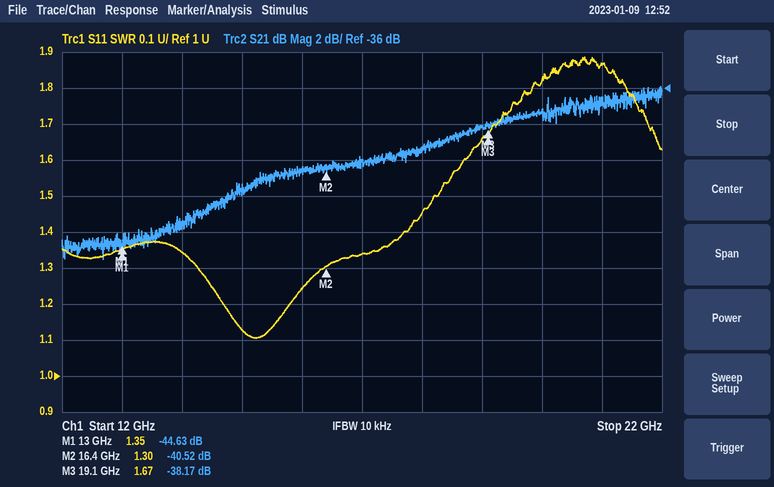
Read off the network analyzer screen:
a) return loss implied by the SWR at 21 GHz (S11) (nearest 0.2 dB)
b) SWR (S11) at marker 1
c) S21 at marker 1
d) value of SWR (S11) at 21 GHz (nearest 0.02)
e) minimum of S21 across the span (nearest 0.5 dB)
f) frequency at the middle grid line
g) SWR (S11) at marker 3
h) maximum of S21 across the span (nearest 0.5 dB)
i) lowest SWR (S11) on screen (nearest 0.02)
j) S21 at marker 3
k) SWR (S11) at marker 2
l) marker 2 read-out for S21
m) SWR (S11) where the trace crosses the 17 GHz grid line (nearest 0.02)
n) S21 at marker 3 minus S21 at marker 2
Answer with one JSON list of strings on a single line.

["10.4 dB", "1.35", "-44.63 dB", "1.86", "-45.5 dB", "17 GHz", "1.67", "-36.0 dB", "1.10", "-38.17 dB", "1.30", "-40.52 dB", "1.34", "2.35 dB"]
